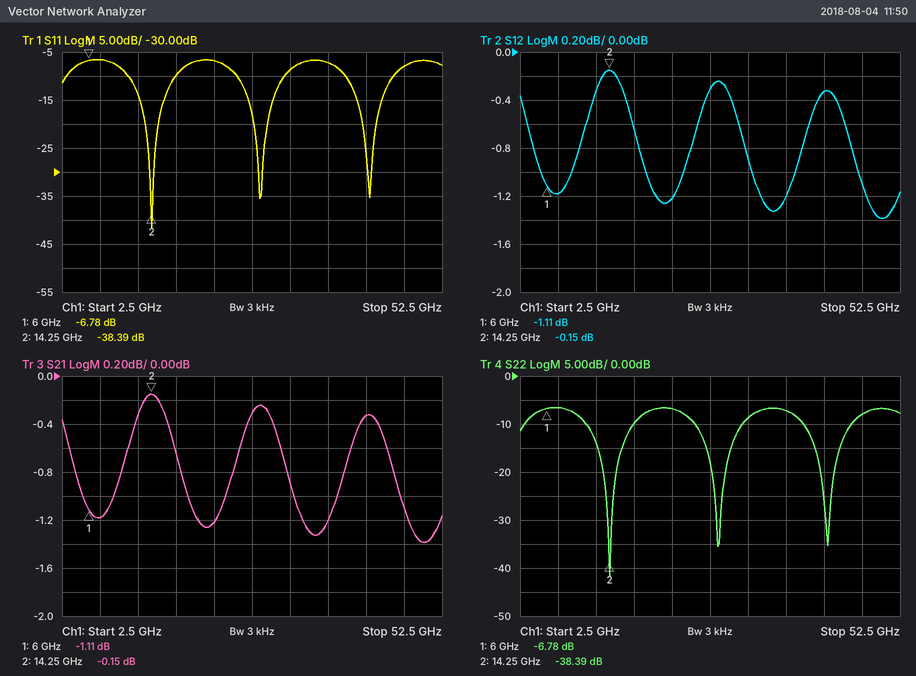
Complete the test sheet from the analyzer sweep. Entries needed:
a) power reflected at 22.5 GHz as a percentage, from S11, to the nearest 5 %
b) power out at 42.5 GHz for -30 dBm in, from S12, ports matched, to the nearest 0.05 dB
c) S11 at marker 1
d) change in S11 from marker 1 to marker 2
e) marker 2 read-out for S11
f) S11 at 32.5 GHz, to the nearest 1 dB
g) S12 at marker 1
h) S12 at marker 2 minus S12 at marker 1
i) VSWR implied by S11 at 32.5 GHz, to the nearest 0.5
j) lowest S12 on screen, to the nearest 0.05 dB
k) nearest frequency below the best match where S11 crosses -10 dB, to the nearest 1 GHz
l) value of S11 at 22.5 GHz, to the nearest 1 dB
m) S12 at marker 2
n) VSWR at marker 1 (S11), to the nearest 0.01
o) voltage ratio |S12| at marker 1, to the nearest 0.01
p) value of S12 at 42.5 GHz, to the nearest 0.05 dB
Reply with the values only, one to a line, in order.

20 %
-30.35 dBm
-6.78 dB
-31.61 dB
-38.39 dB
-9 dB
-1.11 dB
0.96 dB
2.0
-1.40 dB
11 GHz
-7 dB
-0.15 dB
2.69
0.88
-0.35 dB
